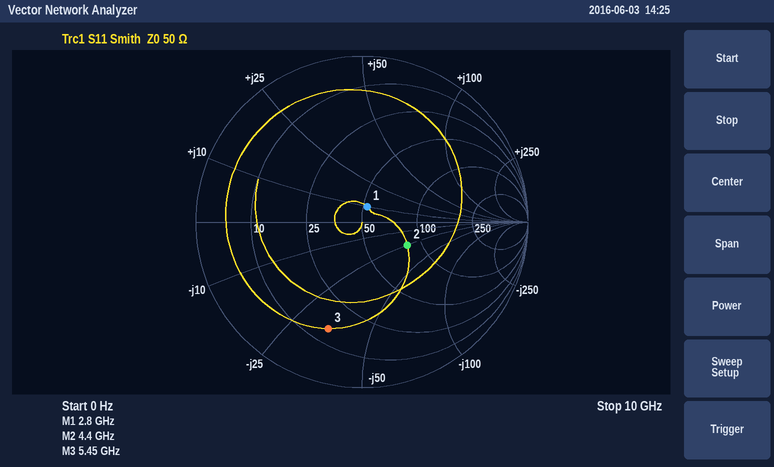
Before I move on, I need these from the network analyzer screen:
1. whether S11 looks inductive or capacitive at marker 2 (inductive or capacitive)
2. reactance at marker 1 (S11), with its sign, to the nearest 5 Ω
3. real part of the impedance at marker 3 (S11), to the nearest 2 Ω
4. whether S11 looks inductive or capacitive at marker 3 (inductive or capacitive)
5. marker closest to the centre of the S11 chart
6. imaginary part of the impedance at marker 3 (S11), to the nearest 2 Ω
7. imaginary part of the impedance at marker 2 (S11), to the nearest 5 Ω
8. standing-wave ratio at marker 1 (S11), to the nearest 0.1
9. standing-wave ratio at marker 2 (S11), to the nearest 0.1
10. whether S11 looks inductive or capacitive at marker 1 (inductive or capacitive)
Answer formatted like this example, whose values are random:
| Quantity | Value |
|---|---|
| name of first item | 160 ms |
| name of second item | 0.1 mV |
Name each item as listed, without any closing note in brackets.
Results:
| Quantity | Value |
|---|---|
| whether S11 looks inductive or capacitive at marker 2 | capacitive |
| reactance at marker 1 (S11), with its sign, to the nearest 5 Ω | +10 Ω |
| real part of the impedance at marker 3 (S11), to the nearest 2 Ω | 14 Ω |
| whether S11 looks inductive or capacitive at marker 3 | capacitive |
| marker closest to the centre of the S11 chart | marker 1 |
| imaginary part of the impedance at marker 3 (S11), to the nearest 2 Ω | -34 Ω |
| imaginary part of the impedance at marker 2 (S11), to the nearest 5 Ω | -25 Ω |
| standing-wave ratio at marker 1 (S11), to the nearest 0.1 | 1.2 |
| standing-wave ratio at marker 2 (S11), to the nearest 0.1 | 1.9 |
| whether S11 looks inductive or capacitive at marker 1 | inductive |
